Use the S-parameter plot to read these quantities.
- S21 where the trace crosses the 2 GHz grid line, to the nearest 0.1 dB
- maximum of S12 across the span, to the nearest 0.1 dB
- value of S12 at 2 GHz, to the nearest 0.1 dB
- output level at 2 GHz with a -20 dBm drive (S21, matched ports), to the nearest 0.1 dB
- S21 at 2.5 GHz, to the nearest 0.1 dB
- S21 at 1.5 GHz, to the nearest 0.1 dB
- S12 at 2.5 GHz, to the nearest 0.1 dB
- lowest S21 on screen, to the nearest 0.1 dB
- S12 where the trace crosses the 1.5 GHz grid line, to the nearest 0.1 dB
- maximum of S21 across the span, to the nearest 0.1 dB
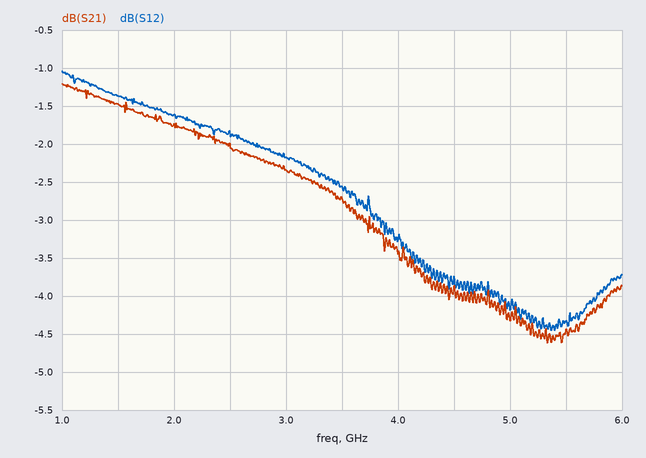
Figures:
-1.7 dB
-1.0 dB
-1.6 dB
-21.7 dBm
-2.0 dB
-1.5 dB
-1.9 dB
-4.6 dB
-1.4 dB
-1.2 dB
